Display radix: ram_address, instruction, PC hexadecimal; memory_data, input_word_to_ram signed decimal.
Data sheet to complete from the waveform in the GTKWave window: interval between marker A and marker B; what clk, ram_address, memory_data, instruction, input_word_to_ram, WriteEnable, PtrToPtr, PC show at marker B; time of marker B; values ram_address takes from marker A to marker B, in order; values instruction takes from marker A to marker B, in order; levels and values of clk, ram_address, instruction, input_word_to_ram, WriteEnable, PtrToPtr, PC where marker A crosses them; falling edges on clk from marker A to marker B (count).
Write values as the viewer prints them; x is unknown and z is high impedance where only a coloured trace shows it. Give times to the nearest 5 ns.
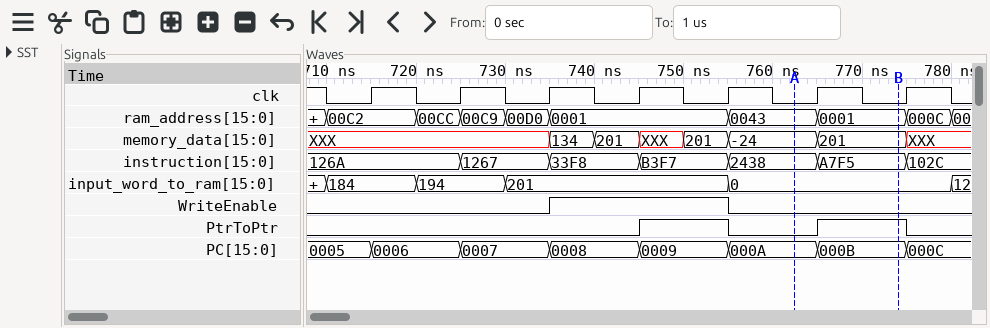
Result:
10 ns
clk=0, ram_address=0001, memory_data=201, instruction=A7F5, input_word_to_ram=0, WriteEnable=0, PtrToPtr=1, PC=000B
775 ns
0043, 0001
2438, A7F5
clk=0, ram_address=0043, instruction=2438, input_word_to_ram=0, WriteEnable=0, PtrToPtr=0, PC=000A
1
